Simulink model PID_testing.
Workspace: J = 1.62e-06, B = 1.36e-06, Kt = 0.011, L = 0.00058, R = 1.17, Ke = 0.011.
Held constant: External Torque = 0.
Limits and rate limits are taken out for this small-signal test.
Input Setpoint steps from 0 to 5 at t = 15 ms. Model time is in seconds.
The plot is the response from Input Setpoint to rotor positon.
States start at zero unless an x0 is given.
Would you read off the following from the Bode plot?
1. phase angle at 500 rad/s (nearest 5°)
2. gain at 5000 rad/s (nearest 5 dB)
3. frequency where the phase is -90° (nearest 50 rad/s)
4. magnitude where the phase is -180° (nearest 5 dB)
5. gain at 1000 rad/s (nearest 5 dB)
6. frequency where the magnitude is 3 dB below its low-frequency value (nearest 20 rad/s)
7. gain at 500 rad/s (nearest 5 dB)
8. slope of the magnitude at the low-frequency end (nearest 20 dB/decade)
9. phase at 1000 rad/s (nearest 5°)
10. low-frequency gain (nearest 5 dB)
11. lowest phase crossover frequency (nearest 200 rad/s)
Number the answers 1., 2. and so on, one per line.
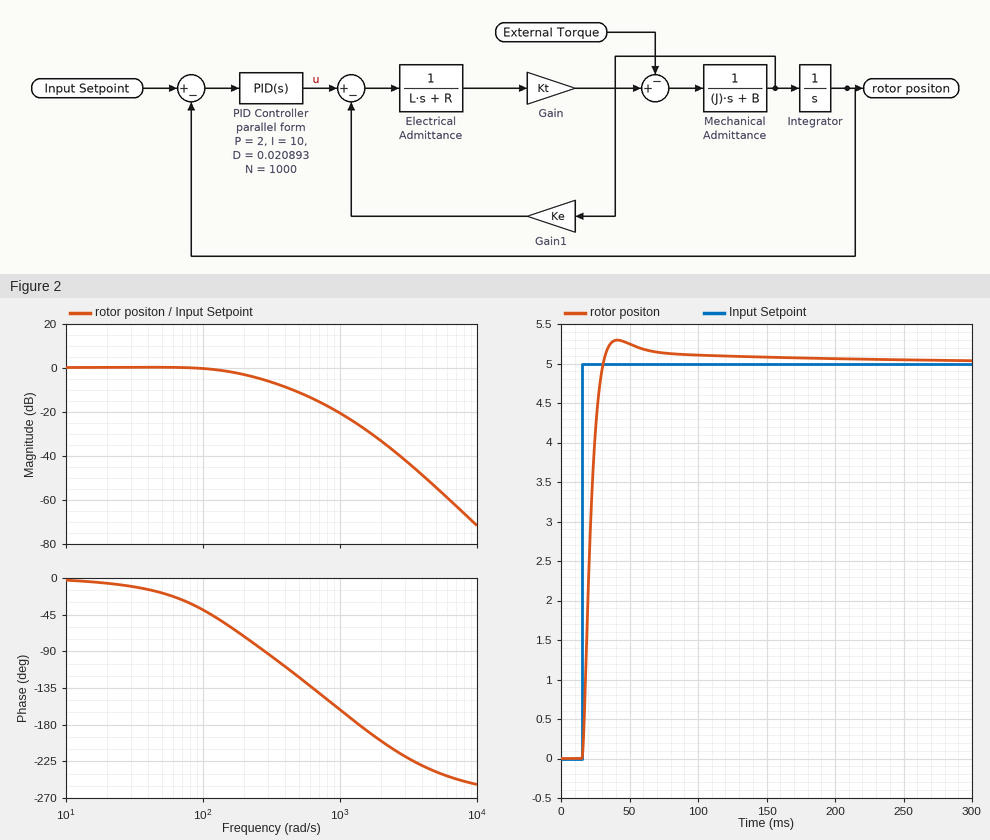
1. -120°
2. -55 dB
3. 300 rad/s
4. -25 dB
5. -20 dB
6. 200 rad/s
7. -10 dB
8. 0 dB/decade
9. -160°
10. 0 dB
11. 1400 rad/s
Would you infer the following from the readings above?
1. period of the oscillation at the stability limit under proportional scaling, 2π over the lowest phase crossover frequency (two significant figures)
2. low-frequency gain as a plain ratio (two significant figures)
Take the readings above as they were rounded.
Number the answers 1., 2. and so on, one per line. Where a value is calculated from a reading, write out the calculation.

1. 2π / 1400 = 0.0045 s
2. 10^(0 / 20) = 1.0
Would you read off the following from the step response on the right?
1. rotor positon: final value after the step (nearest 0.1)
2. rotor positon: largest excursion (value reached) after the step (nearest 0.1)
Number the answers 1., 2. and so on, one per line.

1. 5.0
2. 5.3
